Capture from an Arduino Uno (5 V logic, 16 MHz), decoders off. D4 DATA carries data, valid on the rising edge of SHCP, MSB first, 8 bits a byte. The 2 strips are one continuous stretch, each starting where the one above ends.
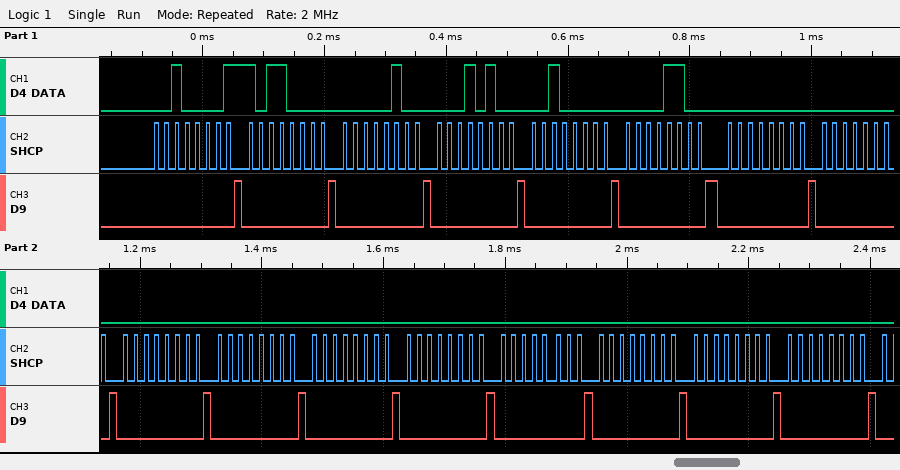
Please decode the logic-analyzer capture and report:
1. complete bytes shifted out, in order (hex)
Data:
21 B0 04 14 20 0C 00 00 00 00 00 00 00 00 00 00
